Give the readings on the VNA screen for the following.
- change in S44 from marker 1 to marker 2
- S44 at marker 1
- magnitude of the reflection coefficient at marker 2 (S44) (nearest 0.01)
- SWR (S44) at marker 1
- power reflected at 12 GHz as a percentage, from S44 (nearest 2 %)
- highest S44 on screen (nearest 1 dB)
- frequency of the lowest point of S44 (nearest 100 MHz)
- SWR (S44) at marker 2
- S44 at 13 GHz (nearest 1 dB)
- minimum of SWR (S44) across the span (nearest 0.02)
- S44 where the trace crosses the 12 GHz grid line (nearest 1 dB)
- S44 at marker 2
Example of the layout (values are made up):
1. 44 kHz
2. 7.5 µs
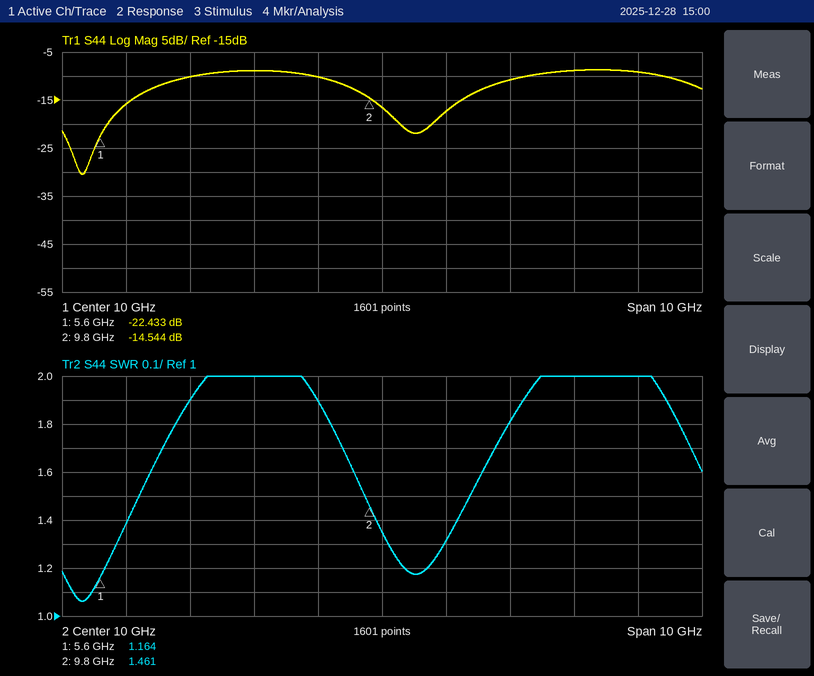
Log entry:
1. 7.889 dB
2. -22.433 dB
3. 0.19
4. 1.164
5. 8 %
6. -9 dB
7. 5.3 GHz
8. 1.461
9. -9 dB
10. 1.06
11. -11 dB
12. -14.544 dB
